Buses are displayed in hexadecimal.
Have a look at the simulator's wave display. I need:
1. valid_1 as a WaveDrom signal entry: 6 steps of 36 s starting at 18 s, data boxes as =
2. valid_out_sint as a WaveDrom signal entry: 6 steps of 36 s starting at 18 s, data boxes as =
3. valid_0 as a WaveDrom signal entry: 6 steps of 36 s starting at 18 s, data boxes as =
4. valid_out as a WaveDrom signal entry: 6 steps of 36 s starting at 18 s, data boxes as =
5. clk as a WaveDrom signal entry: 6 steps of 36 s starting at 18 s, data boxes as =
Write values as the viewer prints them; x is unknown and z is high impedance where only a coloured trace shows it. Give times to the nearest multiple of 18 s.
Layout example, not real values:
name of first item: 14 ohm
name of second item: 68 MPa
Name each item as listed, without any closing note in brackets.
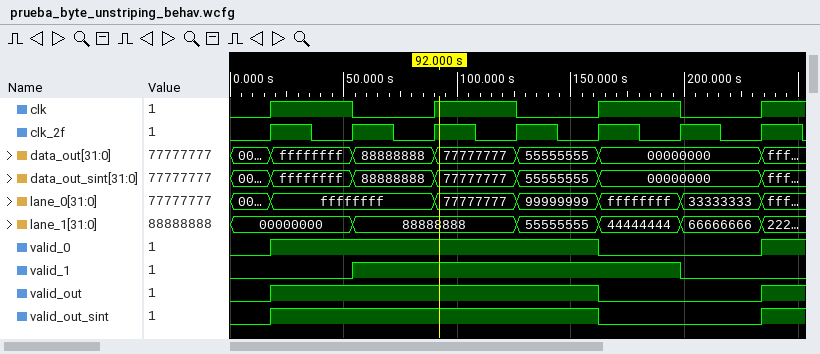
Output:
valid_1 as a WaveDrom signal entry: 6 steps of 36 s starting at 18 s, data boxes as =: {name: 'valid_1', wave: '01...0'}
valid_out_sint as a WaveDrom signal entry: 6 steps of 36 s starting at 18 s, data boxes as =: {name: 'valid_out_sint', wave: '1...0.'}
valid_0 as a WaveDrom signal entry: 6 steps of 36 s starting at 18 s, data boxes as =: {name: 'valid_0', wave: '1...0.'}
valid_out as a WaveDrom signal entry: 6 steps of 36 s starting at 18 s, data boxes as =: {name: 'valid_out', wave: '1...0.'}
clk as a WaveDrom signal entry: 6 steps of 36 s starting at 18 s, data boxes as =: {name: 'clk', wave: '101010'}
